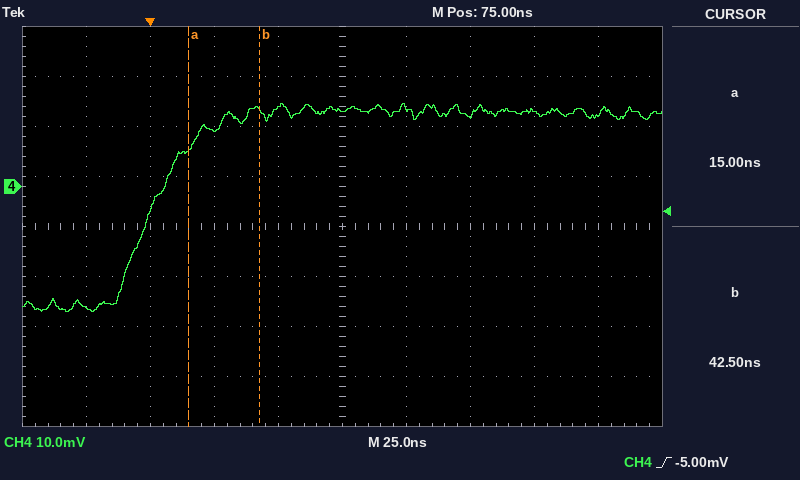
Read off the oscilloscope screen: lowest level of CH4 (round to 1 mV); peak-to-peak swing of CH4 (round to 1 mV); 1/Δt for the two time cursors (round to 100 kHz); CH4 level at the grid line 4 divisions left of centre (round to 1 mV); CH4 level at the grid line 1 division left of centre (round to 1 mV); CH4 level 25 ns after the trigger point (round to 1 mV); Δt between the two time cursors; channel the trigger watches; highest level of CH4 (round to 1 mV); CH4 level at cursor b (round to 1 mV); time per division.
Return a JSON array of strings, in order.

["-25 mV", "42 mV", "36.4 MHz", "-24 mV", "16 mV", "11 mV", "27.5 ns", "CH4", "17 mV", "15 mV", "25 ns"]
